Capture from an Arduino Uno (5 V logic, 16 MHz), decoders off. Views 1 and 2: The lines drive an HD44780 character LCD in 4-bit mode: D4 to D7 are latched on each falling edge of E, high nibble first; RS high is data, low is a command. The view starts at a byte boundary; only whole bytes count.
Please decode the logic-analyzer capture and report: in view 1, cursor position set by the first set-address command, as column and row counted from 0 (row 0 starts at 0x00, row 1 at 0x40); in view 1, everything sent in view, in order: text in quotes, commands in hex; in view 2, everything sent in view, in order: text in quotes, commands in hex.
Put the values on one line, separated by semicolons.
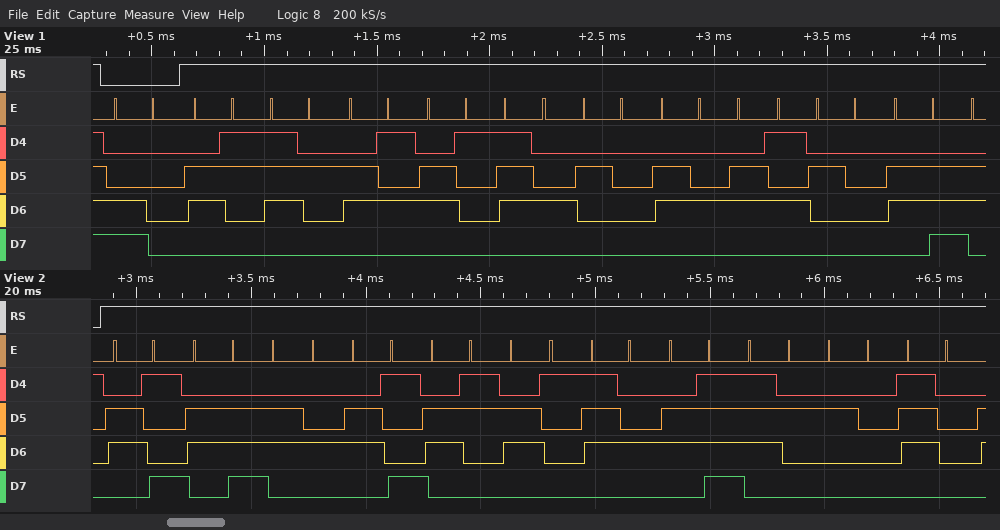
column 0, row 1; 0xC0 "creat de n"; "indicator p"
